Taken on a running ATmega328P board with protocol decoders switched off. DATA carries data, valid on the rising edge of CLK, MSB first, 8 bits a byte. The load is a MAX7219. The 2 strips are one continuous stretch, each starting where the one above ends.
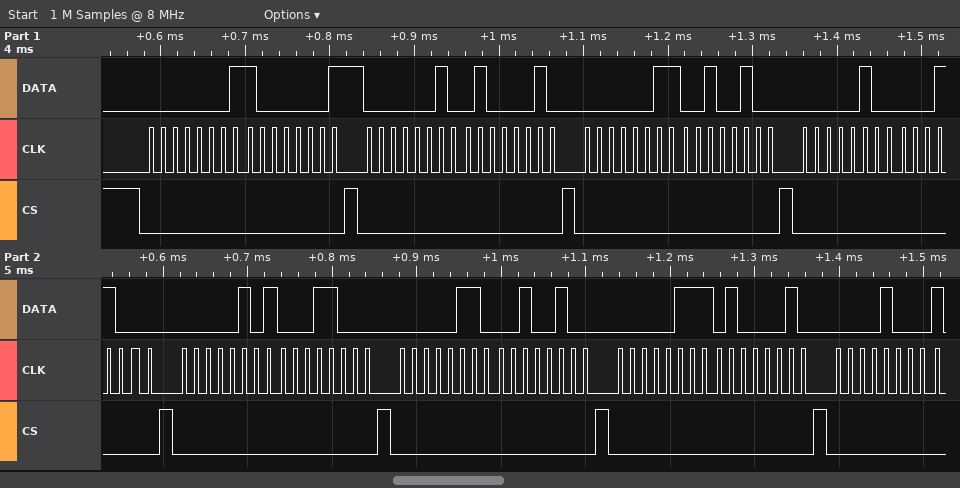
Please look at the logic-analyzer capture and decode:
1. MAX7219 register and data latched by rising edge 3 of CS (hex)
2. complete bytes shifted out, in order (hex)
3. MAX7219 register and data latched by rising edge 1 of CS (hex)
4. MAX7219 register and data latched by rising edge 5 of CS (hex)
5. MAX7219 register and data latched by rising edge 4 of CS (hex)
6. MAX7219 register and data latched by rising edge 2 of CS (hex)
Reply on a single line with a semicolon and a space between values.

register 0x3, data 0x24; 01 81 02 42 03 24 04 18 05 18 06 24 07 42 08; register 0x1, data 0x81; register 0x5, data 0x18; register 0x4, data 0x18; register 0x2, data 0x42
